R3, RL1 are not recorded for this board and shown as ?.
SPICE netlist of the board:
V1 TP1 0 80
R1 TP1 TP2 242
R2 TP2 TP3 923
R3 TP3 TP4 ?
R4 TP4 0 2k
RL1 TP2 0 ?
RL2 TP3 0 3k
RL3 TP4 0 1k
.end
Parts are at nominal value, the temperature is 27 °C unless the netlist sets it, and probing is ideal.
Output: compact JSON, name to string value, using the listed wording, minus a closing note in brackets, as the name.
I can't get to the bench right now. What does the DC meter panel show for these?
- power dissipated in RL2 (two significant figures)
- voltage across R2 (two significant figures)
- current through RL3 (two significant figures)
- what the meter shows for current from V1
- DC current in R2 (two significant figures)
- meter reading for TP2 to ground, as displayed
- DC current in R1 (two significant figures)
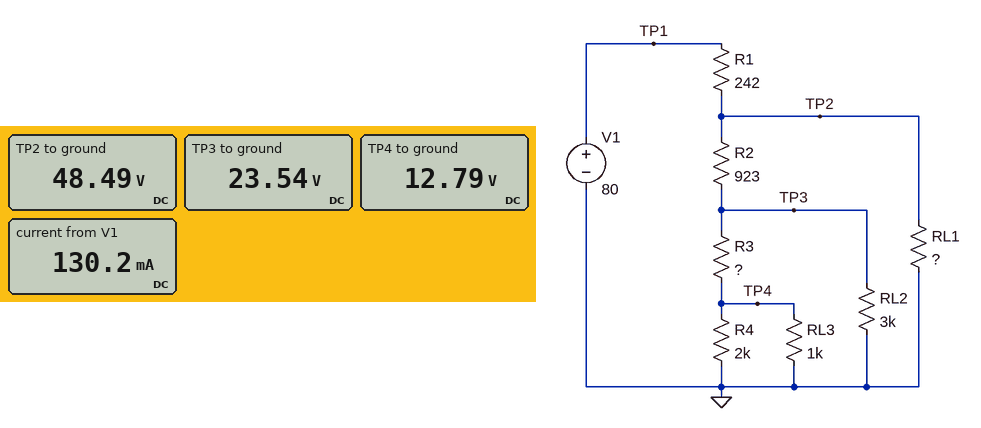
{"power dissipated in RL2": "180 mW", "voltage across R2": "25 V", "current through RL3": "13 mA", "what the meter shows for current from V1": "130.2 mA", "DC current in R2": "27 mA", "meter reading for TP2 to ground, as displayed": "48.49 V", "DC current in R1": "130 mA"}
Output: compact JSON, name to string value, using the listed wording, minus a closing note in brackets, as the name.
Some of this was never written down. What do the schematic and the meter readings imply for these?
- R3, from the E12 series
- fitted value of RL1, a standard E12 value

{"R3, from the E12 series": "560 Ω", "fitted value of RL1, a standard E12 value": "470 Ω"}
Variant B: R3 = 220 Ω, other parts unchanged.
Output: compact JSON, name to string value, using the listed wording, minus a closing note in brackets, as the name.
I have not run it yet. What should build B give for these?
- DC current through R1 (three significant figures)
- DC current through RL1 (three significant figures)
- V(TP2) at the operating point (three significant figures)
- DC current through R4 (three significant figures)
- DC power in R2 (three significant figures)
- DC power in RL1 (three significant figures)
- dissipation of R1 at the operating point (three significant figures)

{"DC current through R1": "132 mA", "DC current through RL1": "102 mA", "V(TP2) at the operating point": "48.0 V", "DC current through R4": "7.69 mA", "DC power in R2": "824 mW", "DC power in RL1": "4.91 W", "dissipation of R1 at the operating point": "4.22 W"}
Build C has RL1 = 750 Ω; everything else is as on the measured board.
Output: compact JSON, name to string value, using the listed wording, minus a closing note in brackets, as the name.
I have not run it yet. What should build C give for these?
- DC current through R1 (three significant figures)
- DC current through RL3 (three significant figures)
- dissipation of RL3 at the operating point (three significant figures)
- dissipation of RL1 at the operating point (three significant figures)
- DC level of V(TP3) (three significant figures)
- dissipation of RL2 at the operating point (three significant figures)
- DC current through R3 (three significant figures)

{"DC current through R1": "104 mA", "DC current through RL3": "14.5 mA", "dissipation of RL3 at the operating point": "210 mW", "dissipation of RL1 at the operating point": "4.02 W", "DC level of V(TP3)": "26.6 V", "dissipation of RL2 at the operating point": "237 mW", "DC current through R3": "21.7 mA"}
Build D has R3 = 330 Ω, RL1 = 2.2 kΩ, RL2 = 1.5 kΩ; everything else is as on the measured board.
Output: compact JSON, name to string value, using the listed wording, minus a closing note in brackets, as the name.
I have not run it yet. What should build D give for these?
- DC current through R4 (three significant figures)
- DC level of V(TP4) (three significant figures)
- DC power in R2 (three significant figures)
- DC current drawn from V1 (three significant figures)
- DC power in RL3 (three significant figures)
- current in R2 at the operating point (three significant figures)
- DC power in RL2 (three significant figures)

{"DC current through R4": "8.30 mA", "DC level of V(TP4)": "16.6 V", "DC power in R2": "1.58 W", "DC current drawn from V1": "70.1 mA", "DC power in RL3": "275 mW", "current in R2 at the operating point": "41.4 mA", "DC power in RL2": "410 mW"}
